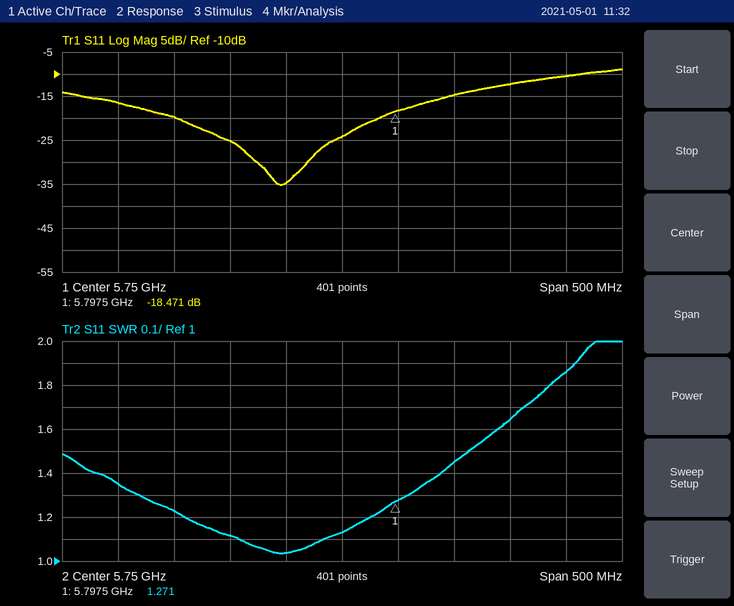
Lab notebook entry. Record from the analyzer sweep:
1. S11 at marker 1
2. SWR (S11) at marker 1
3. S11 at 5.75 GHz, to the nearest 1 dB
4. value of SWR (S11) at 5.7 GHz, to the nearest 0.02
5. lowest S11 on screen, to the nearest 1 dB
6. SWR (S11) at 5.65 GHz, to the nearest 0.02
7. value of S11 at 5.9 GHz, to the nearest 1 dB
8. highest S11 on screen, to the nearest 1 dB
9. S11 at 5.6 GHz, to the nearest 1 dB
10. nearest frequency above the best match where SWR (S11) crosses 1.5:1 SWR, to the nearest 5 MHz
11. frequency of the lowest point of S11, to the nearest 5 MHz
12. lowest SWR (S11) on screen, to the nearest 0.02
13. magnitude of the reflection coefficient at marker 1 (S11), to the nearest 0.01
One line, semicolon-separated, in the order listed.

-18.471 dB; 1.271; -24 dB; 1.04; -35 dB; 1.12; -12 dB; -9 dB; -20 dB; 5.865 GHz; 5.695 GHz; 1.04; 0.12
